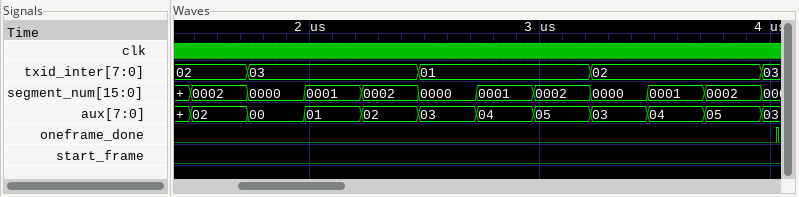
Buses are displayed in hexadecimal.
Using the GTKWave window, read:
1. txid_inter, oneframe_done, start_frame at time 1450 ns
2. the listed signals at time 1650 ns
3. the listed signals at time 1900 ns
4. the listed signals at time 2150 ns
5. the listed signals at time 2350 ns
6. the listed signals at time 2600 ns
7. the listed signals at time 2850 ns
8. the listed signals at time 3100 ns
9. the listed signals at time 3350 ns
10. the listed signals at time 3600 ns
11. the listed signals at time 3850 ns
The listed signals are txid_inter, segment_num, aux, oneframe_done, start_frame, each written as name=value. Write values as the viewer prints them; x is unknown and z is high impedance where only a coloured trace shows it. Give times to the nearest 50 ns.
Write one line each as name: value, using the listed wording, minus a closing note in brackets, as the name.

txid_inter, oneframe_done, start_frame at time 1450 ns: txid_inter=02, oneframe_done=0, start_frame=0
the listed signals at time 1650 ns: txid_inter=02, segment_num=0002, aux=02, oneframe_done=0, start_frame=0
the listed signals at time 1900 ns: txid_inter=03, segment_num=0000, aux=00, oneframe_done=0, start_frame=0
the listed signals at time 2150 ns: txid_inter=03, segment_num=0001, aux=01, oneframe_done=0, start_frame=0
the listed signals at time 2350 ns: txid_inter=03, segment_num=0002, aux=02, oneframe_done=0, start_frame=0
the listed signals at time 2600 ns: txid_inter=01, segment_num=0000, aux=03, oneframe_done=0, start_frame=0
the listed signals at time 2850 ns: txid_inter=01, segment_num=0001, aux=04, oneframe_done=0, start_frame=0
the listed signals at time 3100 ns: txid_inter=01, segment_num=0002, aux=05, oneframe_done=0, start_frame=0
the listed signals at time 3350 ns: txid_inter=02, segment_num=0000, aux=03, oneframe_done=0, start_frame=0
the listed signals at time 3600 ns: txid_inter=02, segment_num=0001, aux=04, oneframe_done=0, start_frame=0
the listed signals at time 3850 ns: txid_inter=02, segment_num=0002, aux=05, oneframe_done=0, start_frame=0
